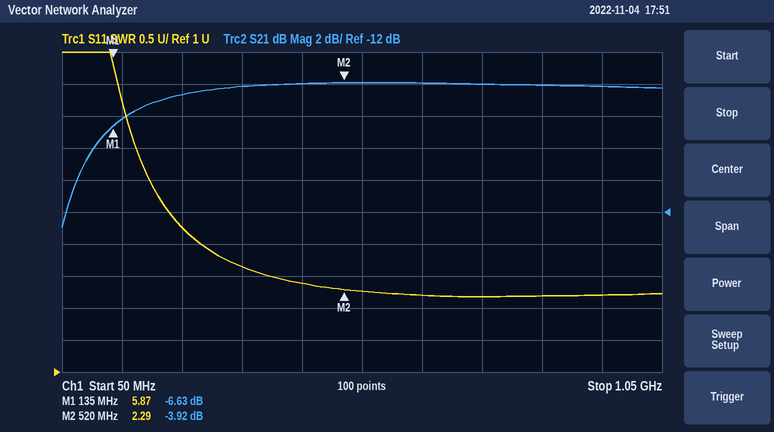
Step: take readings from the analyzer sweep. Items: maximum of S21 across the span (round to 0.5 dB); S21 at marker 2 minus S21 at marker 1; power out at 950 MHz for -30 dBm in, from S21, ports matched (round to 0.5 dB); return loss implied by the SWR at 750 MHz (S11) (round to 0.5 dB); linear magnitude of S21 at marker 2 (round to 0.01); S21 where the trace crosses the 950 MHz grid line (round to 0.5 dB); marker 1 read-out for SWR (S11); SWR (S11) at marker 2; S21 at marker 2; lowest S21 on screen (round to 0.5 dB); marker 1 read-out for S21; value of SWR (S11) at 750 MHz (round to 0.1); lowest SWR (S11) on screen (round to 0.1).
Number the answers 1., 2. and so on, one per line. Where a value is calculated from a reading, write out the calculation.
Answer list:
1. -4.0 dB
2. -3.92 − (-6.63) = 2.71 dB
3. -30 dBm + (-4.0 dB) = -34.0 dBm
4. −20 log10((2.2 − 1)/(2.2 + 1)) ≈ 8.5 dB
5. 10^(-3.92/20) ≈ 0.64
6. -4.0 dB
7. 5.87
8. 2.29
9. -3.92 dB
10. -13.0 dB
11. -6.63 dB
12. 2.2
13. 2.2
